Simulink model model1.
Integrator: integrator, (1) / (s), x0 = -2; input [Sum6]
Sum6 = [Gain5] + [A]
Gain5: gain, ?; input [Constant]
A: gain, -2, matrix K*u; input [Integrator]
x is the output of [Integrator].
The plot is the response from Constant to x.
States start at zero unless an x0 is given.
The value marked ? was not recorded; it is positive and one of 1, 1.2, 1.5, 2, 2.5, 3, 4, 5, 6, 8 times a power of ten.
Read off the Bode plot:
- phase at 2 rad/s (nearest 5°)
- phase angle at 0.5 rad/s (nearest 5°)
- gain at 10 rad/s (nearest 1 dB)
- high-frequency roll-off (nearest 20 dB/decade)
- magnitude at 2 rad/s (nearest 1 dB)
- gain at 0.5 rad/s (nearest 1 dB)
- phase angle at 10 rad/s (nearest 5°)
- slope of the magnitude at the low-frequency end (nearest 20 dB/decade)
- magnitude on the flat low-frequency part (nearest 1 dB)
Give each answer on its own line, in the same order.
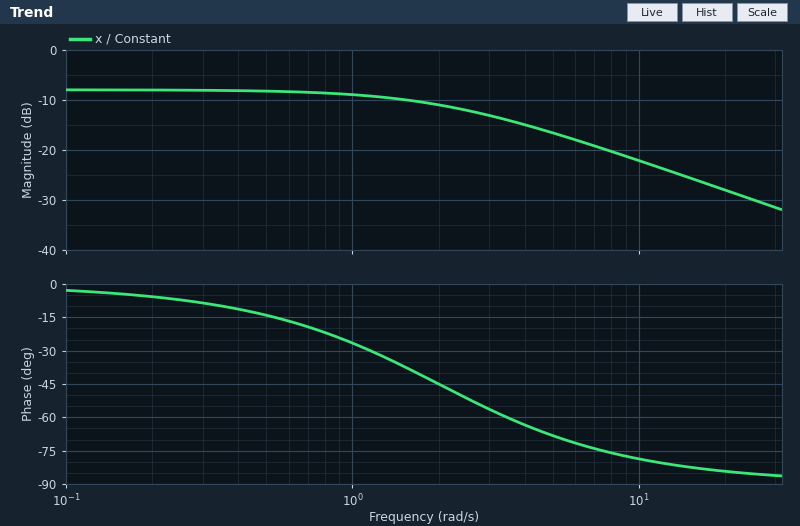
-45°
-15°
-22 dB
-20 dB/decade
-11 dB
-8 dB
-80°
0 dB/decade
-8 dB
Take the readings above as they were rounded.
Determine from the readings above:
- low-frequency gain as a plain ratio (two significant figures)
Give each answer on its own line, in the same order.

0.40
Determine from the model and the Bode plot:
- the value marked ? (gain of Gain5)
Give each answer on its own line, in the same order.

0.8
